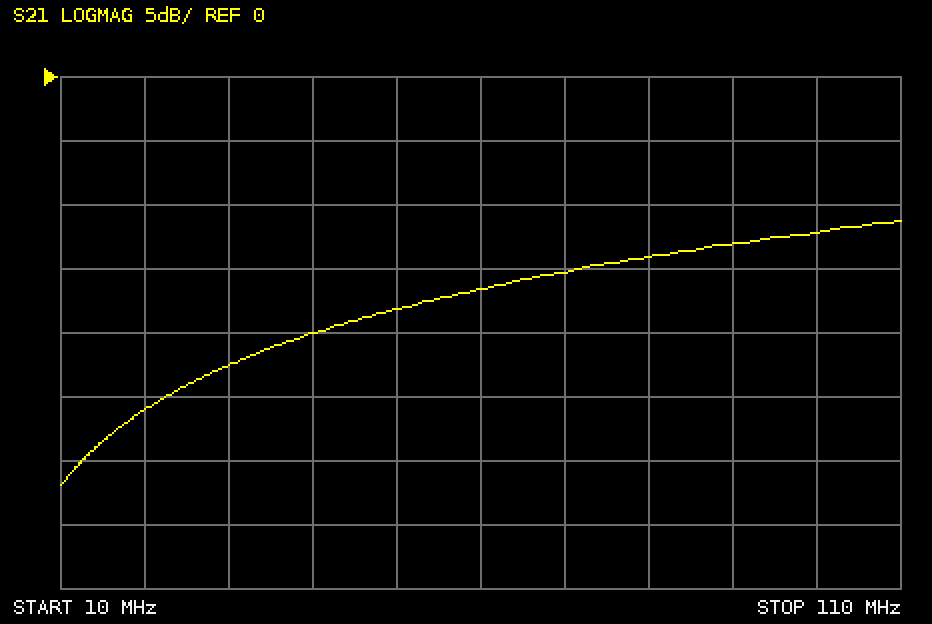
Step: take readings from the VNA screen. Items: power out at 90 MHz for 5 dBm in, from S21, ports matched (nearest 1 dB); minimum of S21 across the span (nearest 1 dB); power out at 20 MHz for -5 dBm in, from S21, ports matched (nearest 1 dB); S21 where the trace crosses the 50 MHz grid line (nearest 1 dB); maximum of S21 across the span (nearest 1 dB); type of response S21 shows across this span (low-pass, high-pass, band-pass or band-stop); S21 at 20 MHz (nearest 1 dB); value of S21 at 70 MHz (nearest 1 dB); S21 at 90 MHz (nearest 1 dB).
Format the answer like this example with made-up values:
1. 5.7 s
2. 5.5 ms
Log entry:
1. -8 dBm
2. -32 dB
3. -31 dBm
4. -18 dB
5. -11 dB
6. high-pass
7. -26 dB
8. -15 dB
9. -13 dB
